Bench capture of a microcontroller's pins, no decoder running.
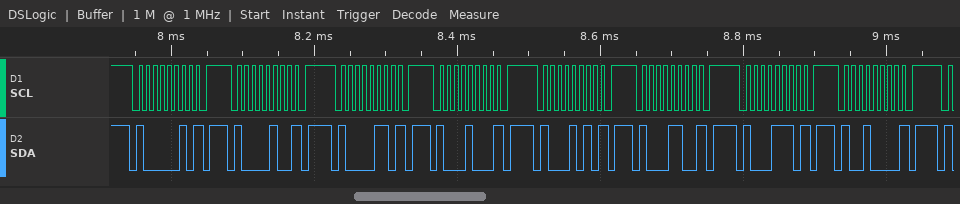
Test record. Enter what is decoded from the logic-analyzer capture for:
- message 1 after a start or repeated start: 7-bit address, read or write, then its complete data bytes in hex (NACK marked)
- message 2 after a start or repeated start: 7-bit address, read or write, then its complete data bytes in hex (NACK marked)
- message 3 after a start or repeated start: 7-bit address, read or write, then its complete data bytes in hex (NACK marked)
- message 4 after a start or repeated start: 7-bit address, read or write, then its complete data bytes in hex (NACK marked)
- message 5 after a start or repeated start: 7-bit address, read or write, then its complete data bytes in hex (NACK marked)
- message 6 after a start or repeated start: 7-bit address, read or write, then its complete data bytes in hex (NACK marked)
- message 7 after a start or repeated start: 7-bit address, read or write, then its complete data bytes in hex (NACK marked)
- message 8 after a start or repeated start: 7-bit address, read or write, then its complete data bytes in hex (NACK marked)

0x41 write NACK
0x42 write NACK
0x43 write NACK
0x44 write NACK
0x45 write NACK
0x46 write NACK
0x47 write NACK
0x48 write NACK
